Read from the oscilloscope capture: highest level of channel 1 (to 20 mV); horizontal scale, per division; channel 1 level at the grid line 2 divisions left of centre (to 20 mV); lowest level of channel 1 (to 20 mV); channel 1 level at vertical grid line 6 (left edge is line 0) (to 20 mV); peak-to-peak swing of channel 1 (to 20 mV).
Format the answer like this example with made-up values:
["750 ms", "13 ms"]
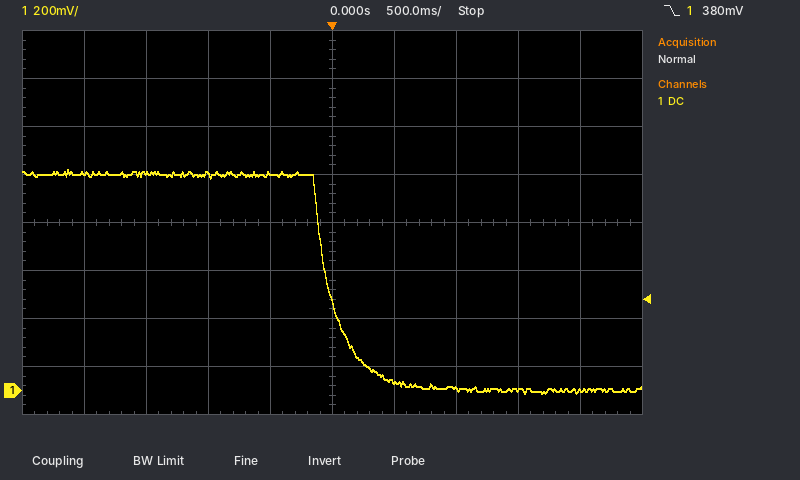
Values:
["920 mV", "500 ms", "900 mV", "-20 mV", "40 mV", "940 mV"]
